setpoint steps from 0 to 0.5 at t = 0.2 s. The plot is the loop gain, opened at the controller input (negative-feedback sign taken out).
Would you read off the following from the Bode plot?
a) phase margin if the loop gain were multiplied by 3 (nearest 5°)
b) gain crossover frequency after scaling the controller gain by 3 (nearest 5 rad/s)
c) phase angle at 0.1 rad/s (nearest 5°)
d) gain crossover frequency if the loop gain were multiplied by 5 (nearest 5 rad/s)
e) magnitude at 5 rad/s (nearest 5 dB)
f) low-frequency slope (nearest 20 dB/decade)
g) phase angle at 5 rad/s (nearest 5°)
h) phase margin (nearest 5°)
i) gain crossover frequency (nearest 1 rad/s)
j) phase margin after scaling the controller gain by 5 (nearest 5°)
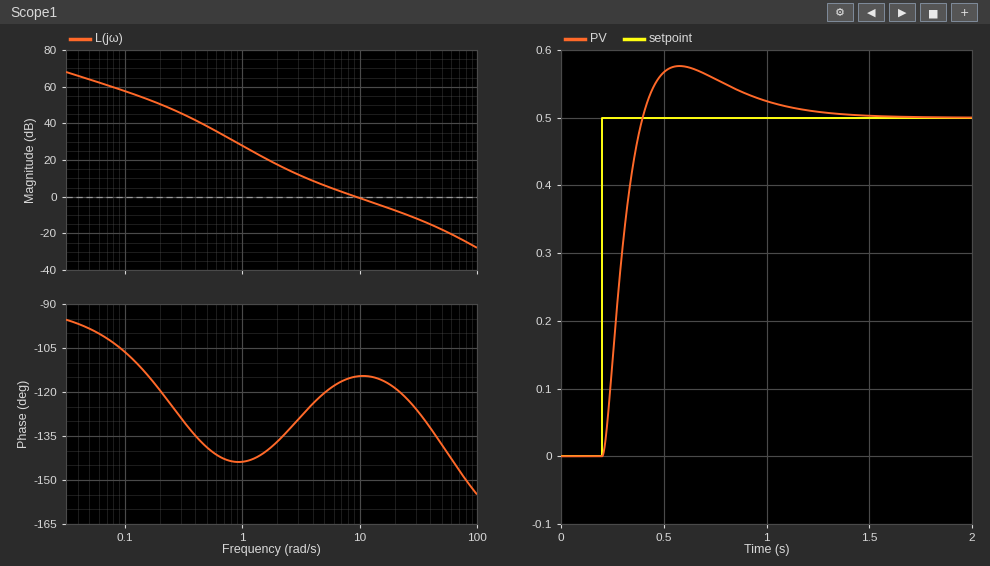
60°
25 rad/s
-105°
35 rad/s
5 dB
-20 dB/decade
-120°
65°
9 rad/s
50°
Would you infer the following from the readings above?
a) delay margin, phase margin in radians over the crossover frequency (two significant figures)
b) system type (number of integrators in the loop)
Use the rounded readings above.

0.13 s
1
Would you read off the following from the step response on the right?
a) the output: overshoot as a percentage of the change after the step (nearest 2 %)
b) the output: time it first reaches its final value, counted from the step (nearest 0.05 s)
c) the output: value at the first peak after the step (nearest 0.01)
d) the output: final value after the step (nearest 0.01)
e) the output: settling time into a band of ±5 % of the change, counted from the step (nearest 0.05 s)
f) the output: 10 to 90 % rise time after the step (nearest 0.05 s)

16 %
0.20 s
0.58
0.50
0.80 s
0.15 s
